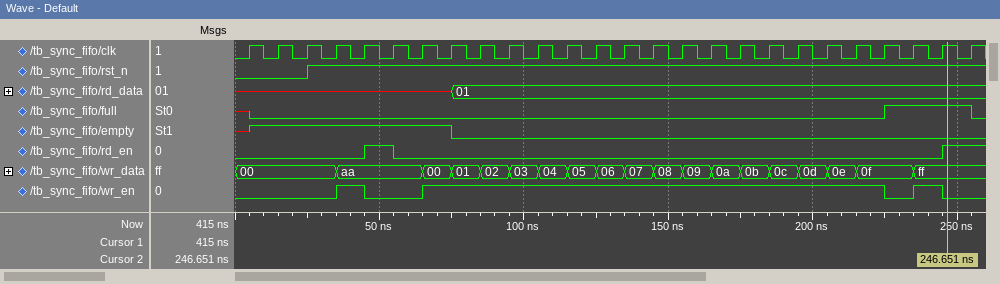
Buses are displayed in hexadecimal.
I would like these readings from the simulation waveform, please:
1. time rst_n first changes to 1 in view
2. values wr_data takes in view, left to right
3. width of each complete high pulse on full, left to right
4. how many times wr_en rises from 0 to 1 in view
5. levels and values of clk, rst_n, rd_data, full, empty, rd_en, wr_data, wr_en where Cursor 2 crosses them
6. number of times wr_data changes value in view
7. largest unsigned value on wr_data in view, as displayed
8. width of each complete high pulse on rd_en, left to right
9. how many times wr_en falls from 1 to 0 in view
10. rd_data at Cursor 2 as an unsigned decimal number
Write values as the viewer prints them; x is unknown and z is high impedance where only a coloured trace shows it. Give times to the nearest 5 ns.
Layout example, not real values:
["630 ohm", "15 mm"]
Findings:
["25 ns", "00, aa, 00, 01, 02, 03, 04, 05, 06, 07, 08, 09, 0a, 0b, 0c, 0d, 0e, 0f, ff", "30 ns", "3", "clk=1, rst_n=1, rd_data=01, full=1, empty=0, rd_en=1, wr_data=ff, wr_en=0", "18", "ff", "10 ns", "3", "1"]
